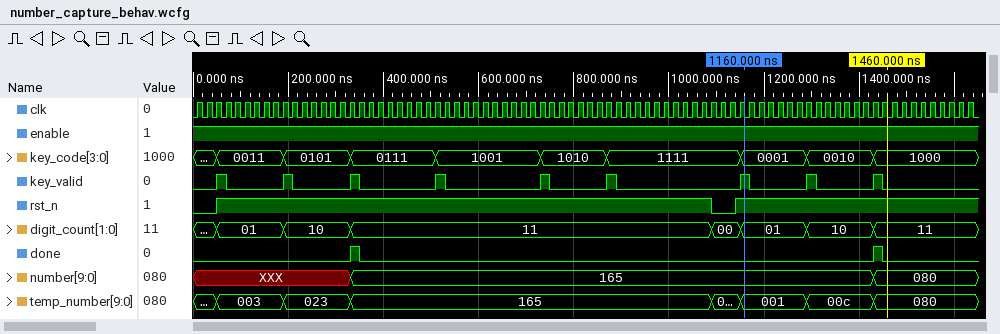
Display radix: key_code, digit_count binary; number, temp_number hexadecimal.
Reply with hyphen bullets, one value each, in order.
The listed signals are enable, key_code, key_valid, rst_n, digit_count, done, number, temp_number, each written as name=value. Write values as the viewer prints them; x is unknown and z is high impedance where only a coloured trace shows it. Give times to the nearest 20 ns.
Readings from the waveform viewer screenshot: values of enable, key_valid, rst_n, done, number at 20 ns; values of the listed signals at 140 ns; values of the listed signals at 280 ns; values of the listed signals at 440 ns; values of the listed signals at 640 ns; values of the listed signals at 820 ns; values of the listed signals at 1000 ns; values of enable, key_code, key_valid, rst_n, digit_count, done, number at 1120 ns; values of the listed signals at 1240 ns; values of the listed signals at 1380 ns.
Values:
- enable=1, key_valid=0, rst_n=0, done=0, number=XXX
- enable=1, key_code=0011, key_valid=0, rst_n=1, digit_count=01, done=0, number=XXX, temp_number=003
- enable=1, key_code=0101, key_valid=0, rst_n=1, digit_count=10, done=0, number=XXX, temp_number=023
- enable=1, key_code=0111, key_valid=0, rst_n=1, digit_count=11, done=0, number=165, temp_number=165
- enable=1, key_code=1001, key_valid=0, rst_n=1, digit_count=11, done=0, number=165, temp_number=165
- enable=1, key_code=1010, key_valid=0, rst_n=1, digit_count=11, done=0, number=165, temp_number=165
- enable=1, key_code=1111, key_valid=0, rst_n=1, digit_count=11, done=0, number=165, temp_number=165
- enable=1, key_code=1111, key_valid=0, rst_n=0, digit_count=00, done=0, number=165
- enable=1, key_code=0001, key_valid=0, rst_n=1, digit_count=01, done=0, number=165, temp_number=001
- enable=1, key_code=0010, key_valid=0, rst_n=1, digit_count=10, done=0, number=165, temp_number=00c
